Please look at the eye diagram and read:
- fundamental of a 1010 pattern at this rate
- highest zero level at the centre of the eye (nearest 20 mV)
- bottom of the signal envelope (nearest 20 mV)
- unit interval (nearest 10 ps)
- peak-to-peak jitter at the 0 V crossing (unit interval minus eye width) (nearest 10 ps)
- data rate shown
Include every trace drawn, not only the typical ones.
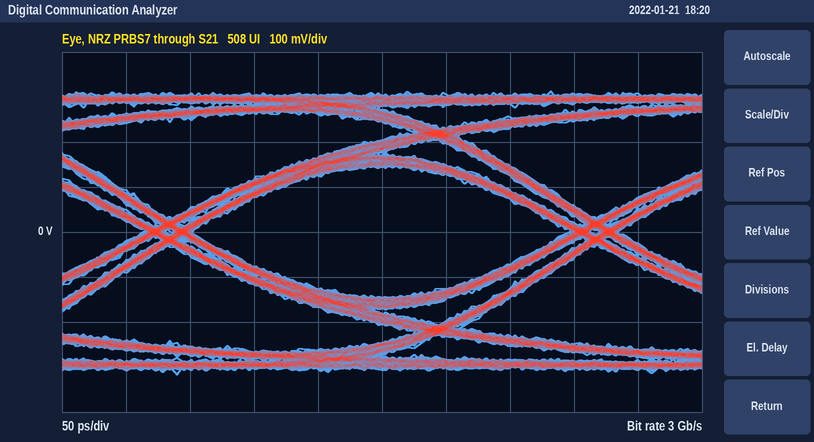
1.5 GHz
-140 mV
-320 mV
330 ps
40 ps
3 Gb/s
